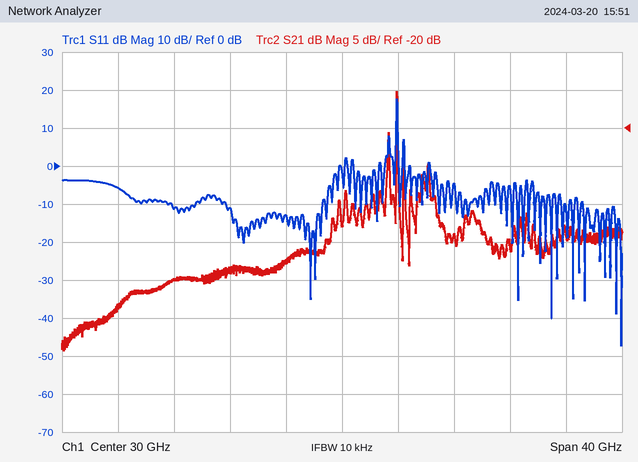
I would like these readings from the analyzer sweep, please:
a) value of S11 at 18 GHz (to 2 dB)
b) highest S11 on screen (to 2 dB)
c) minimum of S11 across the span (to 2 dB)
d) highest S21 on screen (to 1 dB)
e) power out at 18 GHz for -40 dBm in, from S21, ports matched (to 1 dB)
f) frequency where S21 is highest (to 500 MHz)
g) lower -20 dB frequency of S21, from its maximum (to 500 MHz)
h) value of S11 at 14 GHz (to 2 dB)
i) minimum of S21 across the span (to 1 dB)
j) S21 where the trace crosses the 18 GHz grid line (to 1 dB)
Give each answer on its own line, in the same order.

-12 dB
18 dB
-48 dB
-15 dB
-80 dBm
34.0 GHz
29.0 GHz
-6 dB
-49 dB
-40 dB
